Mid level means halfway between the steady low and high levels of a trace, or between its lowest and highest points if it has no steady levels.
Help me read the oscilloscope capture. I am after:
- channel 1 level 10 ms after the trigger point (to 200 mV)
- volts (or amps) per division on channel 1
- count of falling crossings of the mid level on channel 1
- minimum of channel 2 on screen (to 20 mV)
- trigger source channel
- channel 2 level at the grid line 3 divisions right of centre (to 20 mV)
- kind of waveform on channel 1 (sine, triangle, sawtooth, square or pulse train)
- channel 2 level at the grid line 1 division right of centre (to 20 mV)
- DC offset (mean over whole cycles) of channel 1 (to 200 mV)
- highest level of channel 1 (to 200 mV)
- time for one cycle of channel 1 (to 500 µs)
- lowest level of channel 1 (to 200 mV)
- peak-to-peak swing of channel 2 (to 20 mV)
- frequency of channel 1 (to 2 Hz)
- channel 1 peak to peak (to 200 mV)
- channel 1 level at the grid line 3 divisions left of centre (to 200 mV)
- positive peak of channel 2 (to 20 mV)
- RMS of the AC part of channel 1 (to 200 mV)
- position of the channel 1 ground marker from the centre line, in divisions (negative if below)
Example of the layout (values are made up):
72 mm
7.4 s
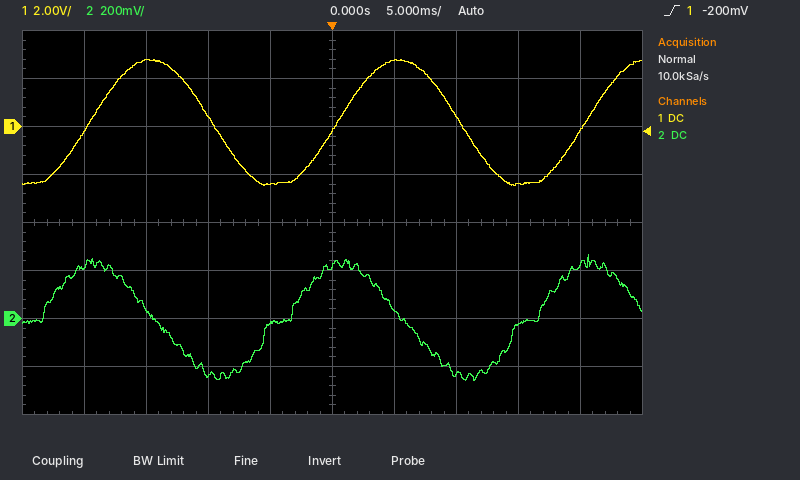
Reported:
400 mV
2 V
2
-260 mV
channel 1
-20 mV
sine
40 mV
200 mV
2.8 V
20.0 ms
-2.4 V
520 mV
50 Hz
5.2 V
2.8 V
260 mV
1.8 V
+2.0 div
